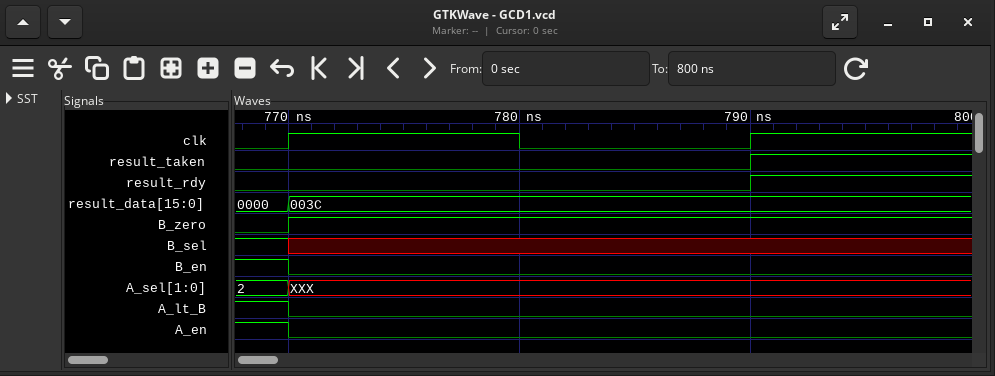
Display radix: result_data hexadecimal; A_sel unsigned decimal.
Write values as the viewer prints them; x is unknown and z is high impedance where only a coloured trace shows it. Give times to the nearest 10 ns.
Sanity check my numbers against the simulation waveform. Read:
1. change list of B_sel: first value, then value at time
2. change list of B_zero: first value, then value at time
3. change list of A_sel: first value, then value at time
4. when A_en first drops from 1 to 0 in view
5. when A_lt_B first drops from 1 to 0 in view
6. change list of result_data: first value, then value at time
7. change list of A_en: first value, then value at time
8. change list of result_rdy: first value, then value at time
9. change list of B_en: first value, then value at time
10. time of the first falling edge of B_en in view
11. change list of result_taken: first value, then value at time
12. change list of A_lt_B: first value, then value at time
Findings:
1, x at 770 ns
0, 1 at 770 ns
2, XXX at 770 ns
770 ns
770 ns
0000, 003C at 770 ns
1, 0 at 770 ns
0, 1 at 790 ns
1, 0 at 770 ns
770 ns
0, 1 at 790 ns
1, 0 at 770 ns
